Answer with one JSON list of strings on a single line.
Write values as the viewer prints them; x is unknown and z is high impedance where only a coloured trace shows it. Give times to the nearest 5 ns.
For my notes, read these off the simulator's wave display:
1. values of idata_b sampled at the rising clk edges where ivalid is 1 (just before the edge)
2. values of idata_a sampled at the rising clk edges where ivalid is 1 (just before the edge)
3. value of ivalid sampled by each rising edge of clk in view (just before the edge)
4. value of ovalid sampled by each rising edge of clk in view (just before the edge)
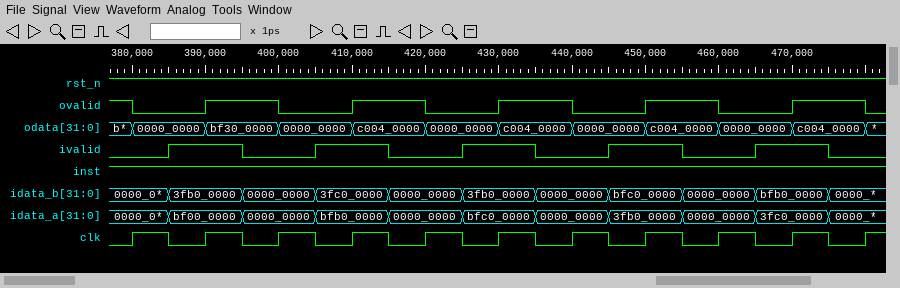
["3fb0_0000, 3fc0_0000, 3fb0_0000, bfc0_0000, bfb0_0000", "bf00_0000, bfb0_0000, bfc0_0000, 3fb0_0000, 3fc0_0000", "0 1 0 1 0 1 0 1 0 1 0", "1 0 1 0 1 0 1 0 1 0 1"]
